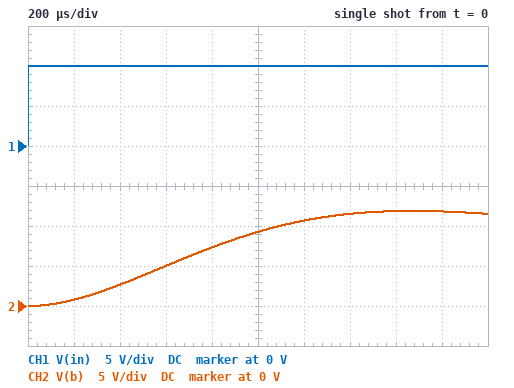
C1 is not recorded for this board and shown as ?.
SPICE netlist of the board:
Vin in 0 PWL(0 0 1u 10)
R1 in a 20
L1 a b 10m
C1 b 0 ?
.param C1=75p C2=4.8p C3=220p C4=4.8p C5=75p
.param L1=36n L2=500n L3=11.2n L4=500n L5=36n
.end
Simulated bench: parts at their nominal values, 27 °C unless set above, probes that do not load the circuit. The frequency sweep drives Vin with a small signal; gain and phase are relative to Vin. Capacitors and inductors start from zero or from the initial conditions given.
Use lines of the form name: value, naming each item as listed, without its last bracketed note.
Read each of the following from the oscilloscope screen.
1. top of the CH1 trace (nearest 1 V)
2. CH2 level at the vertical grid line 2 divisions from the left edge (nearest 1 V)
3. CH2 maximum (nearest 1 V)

top of the CH1 trace: 10 V
CH2 level at the vertical grid line 2 divisions from the left edge: 3 V
CH2 maximum: 12 V
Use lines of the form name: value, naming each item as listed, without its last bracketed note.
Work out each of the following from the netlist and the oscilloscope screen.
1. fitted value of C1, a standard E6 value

fitted value of C1, a standard E6 value: 22 µF
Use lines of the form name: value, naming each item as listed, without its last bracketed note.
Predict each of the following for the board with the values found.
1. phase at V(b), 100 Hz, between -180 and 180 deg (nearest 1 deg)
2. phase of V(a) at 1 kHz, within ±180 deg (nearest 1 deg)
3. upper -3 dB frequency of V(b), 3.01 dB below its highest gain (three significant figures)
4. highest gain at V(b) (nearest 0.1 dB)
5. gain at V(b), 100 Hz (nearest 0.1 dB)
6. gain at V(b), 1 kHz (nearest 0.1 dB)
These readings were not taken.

phase at V(b), 100 Hz, between -180 and 180 deg: -17 deg
phase of V(a) at 1 kHz, within ±180 deg: 20 deg
upper -3 dB frequency of V(b), 3.01 dB below its highest gain: 400 Hz
highest gain at V(b): 1.6 dB
gain at V(b), 100 Hz: 0.4 dB
gain at V(b), 1 kHz: -18.2 dB
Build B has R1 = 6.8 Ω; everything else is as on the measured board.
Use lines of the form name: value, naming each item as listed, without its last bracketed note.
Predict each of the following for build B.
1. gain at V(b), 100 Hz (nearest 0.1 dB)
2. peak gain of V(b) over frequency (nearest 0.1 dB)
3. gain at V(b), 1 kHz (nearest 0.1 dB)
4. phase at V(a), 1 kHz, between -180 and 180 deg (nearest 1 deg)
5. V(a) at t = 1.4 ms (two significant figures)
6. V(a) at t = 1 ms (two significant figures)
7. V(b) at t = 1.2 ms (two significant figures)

gain at V(b), 100 Hz: 0.7 dB
peak gain of V(b) over frequency: 10.0 dB
gain at V(b), 1 kHz: -17.8 dB
phase at V(a), 1 kHz, between -180 and 180 deg: 7 deg
V(a) at t = 1.4 ms: 9.6 V
V(a) at t = 1 ms: 8.0 V
V(b) at t = 1.2 ms: 15 V
